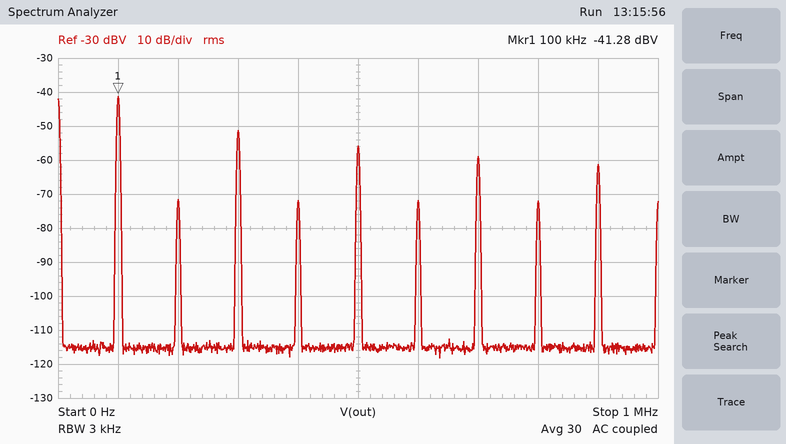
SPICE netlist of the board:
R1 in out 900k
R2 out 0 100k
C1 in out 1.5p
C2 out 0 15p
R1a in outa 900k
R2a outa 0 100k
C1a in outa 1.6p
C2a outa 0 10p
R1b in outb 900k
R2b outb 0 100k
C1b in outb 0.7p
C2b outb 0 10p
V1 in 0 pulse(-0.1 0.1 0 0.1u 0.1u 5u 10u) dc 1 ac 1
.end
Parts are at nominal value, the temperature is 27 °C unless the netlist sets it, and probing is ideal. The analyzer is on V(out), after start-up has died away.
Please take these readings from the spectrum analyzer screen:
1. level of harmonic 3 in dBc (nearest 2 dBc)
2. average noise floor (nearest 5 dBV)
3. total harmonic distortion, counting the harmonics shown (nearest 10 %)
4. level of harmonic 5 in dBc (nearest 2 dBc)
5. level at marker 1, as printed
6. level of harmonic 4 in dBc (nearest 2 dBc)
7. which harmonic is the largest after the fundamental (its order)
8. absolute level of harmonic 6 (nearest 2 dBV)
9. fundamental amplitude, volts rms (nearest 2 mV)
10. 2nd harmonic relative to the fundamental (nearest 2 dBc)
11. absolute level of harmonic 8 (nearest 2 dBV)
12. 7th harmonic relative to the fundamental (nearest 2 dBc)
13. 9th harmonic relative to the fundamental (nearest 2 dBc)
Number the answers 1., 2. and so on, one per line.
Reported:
1. -10 dBc
2. -115 dBV
3. 40 %
4. -14 dBc
5. -41.28 dBV
6. -30 dBc
7. 3
8. -72 dBV
9. 8 mV
10. -30 dBc
11. -72 dBV
12. -18 dBc
13. -20 dBc
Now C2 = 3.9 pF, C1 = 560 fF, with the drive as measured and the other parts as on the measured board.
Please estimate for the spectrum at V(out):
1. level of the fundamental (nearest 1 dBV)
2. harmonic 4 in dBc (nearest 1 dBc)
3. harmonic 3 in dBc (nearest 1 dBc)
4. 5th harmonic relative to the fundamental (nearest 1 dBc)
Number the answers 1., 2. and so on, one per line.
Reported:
1. -41 dBV
2. -29 dBc
3. -9 dBc
4. -13 dBc
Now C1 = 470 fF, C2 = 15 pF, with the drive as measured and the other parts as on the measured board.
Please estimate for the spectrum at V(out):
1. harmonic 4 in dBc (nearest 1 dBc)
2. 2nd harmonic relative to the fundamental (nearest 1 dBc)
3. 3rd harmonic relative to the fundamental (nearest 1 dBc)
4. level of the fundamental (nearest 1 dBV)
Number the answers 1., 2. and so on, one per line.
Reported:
1. -36 dBc
2. -33 dBc
3. -14 dBc
4. -43 dBV
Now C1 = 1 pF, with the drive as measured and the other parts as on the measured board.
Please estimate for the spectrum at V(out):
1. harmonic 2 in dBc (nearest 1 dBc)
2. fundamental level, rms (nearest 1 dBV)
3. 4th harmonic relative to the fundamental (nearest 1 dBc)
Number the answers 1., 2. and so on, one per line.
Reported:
1. -31 dBc
2. -42 dBV
3. -32 dBc
